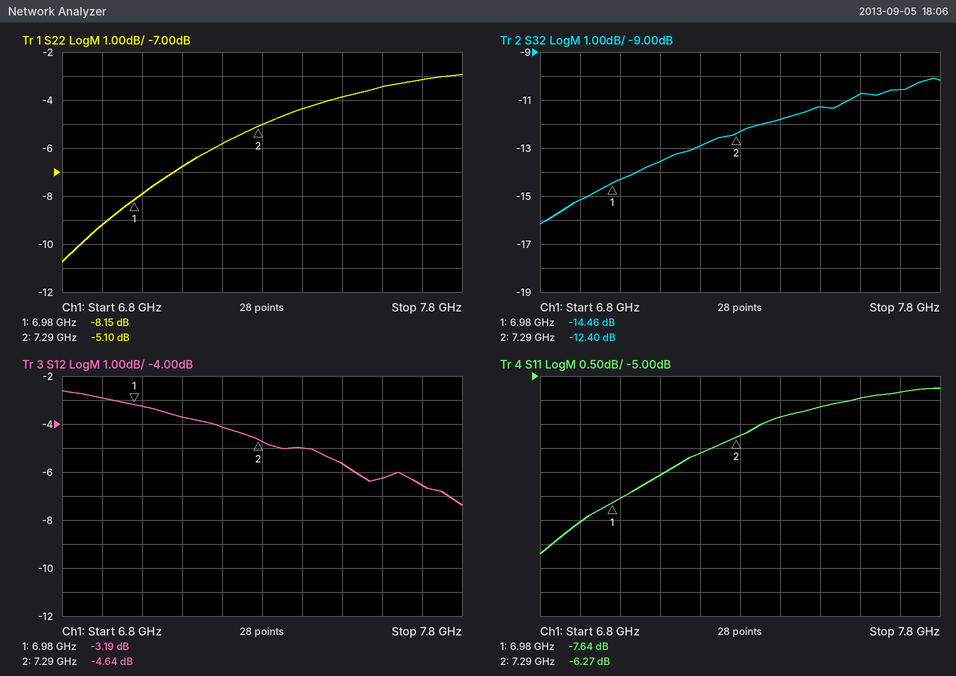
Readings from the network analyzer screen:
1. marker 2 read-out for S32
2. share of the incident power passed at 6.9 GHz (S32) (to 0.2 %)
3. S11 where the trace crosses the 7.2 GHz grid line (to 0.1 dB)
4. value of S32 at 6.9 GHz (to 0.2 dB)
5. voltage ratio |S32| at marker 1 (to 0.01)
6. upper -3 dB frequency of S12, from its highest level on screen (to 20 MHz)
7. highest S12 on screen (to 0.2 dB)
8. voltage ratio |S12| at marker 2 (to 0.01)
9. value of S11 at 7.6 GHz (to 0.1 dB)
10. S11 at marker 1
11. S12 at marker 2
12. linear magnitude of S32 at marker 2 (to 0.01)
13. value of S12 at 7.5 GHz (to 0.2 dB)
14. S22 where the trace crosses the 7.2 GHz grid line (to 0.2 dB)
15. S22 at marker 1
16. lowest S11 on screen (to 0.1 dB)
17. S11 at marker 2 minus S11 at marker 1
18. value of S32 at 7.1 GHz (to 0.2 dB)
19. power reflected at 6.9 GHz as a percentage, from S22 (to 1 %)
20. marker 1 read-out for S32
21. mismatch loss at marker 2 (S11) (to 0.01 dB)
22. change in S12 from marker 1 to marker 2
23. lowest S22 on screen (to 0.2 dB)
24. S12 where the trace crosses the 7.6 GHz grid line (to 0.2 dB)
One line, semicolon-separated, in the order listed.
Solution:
-12.40 dB; 3.0 %; -6.6 dB; -15.2 dB; 0.19; 7.50 GHz; -2.6 dB; 0.59; -5.5 dB; -7.64 dB; -4.64 dB; 0.24; -5.6 dB; -5.8 dB; -8.15 dB; -8.7 dB; 1.37 dB; -13.6 dB; 12 %; -14.46 dB; 1.17 dB; -1.45 dB; -10.8 dB; -6.2 dB
